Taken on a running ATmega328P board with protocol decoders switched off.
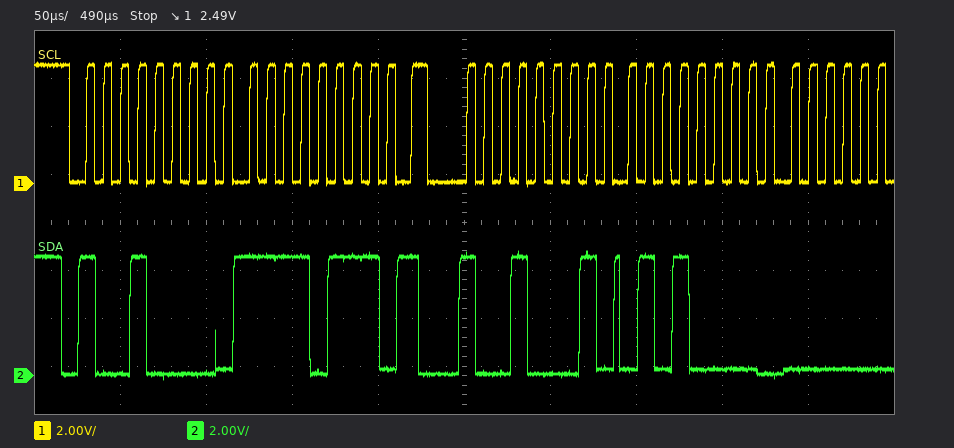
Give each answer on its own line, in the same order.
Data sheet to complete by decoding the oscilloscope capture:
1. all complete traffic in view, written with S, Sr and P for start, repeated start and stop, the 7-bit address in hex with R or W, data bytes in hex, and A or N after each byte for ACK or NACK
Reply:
S 48W A F7 A Sr 48R A 50 A
